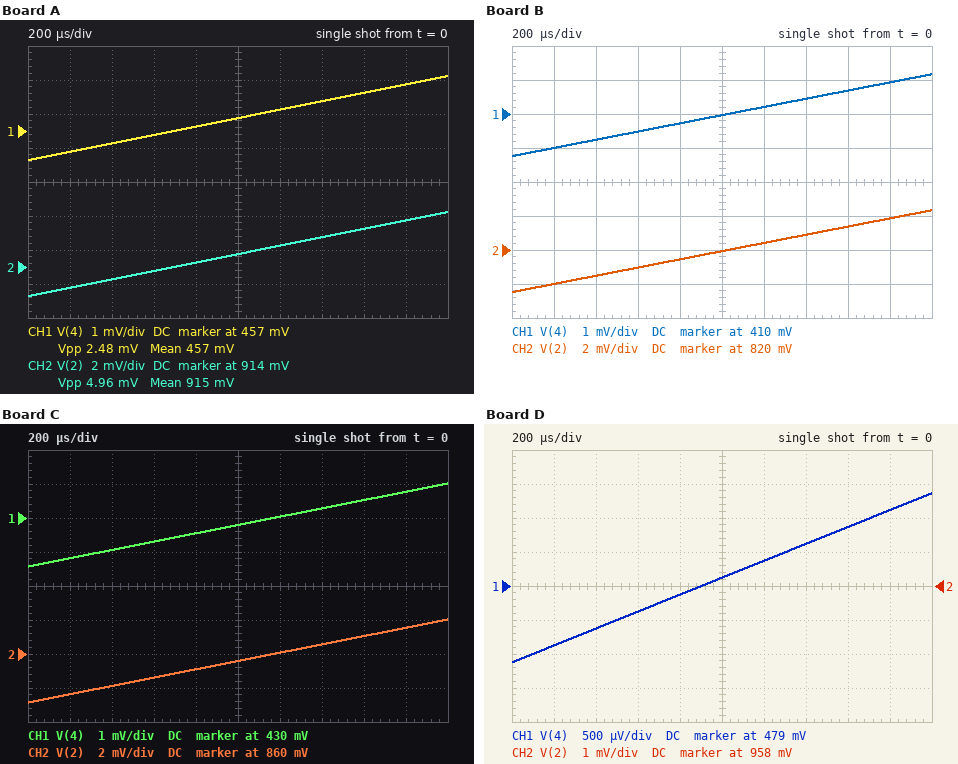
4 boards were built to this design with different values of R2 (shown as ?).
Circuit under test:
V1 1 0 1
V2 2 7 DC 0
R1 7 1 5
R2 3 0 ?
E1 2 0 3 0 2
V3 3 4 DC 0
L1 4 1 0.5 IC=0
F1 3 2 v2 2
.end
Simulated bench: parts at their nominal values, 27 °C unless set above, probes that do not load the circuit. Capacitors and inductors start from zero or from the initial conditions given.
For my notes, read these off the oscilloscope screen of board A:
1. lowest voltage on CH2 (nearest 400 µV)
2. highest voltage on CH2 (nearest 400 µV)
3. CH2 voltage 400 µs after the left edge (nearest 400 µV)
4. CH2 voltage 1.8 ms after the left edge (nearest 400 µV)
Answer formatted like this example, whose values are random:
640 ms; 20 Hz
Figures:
912.4 mV; 917.2 mV; 913.2 mV; 916.8 mV
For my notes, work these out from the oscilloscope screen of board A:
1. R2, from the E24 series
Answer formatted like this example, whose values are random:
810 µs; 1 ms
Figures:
13 Ω
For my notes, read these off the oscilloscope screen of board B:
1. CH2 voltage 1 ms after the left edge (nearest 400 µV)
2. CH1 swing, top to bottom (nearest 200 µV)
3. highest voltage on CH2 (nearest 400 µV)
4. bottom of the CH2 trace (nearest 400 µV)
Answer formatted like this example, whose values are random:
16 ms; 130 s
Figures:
820.0 mV; 2.4 mV; 822.4 mV; 817.6 mV
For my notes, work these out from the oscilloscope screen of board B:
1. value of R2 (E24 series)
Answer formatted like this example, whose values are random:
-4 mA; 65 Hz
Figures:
5.6 Ω
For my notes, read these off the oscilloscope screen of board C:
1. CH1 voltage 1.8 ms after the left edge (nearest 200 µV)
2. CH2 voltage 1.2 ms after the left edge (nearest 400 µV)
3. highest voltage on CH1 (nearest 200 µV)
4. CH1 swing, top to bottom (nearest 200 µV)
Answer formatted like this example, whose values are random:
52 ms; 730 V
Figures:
430.8 mV; 860.0 mV; 431.0 mV; 2.4 mV
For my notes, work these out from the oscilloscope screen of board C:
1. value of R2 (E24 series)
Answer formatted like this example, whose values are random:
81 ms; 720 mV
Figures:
7.5 Ω
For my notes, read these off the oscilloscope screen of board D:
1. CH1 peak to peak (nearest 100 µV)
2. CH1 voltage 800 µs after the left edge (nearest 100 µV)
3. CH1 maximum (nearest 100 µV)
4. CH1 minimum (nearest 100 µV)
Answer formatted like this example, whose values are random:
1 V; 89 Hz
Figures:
2.5 mV; 478.9 mV; 480.4 mV; 477.9 mV
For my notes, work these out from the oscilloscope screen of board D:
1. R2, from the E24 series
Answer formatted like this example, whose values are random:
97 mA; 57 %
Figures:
27 Ω
